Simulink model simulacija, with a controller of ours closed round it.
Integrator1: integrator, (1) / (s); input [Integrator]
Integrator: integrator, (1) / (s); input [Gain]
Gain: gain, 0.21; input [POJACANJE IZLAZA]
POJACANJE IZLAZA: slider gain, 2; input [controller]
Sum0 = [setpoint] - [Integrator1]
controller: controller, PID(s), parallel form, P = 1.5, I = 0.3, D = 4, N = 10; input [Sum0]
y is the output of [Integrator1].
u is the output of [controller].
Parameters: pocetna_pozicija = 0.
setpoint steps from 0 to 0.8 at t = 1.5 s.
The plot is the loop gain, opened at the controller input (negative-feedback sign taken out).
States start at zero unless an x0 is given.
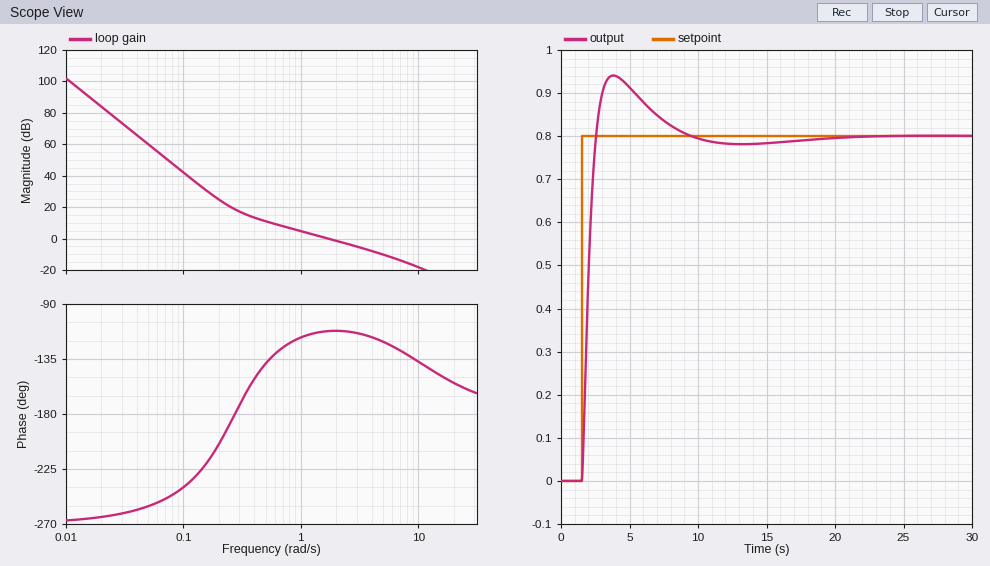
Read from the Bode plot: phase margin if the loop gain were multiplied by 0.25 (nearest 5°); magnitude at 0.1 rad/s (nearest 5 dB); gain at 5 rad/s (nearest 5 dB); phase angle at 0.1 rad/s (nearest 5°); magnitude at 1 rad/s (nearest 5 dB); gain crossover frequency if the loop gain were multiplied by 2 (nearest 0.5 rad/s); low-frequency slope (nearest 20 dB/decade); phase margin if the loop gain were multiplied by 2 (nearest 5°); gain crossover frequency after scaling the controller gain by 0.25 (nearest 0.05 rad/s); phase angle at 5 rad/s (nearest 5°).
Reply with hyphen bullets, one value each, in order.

- 35°
- 40 dB
- -10 dB
- -240°
- 5 dB
- 3.5 rad/s
- -60 dB/decade
- 65°
- 0.45 rad/s
- -120°
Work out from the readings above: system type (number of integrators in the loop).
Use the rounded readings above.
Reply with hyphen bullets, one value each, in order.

- 3
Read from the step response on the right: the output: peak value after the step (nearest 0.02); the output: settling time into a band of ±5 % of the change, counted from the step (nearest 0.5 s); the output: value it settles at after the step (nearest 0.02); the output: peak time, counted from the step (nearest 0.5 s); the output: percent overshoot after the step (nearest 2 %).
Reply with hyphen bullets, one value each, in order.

- 0.94
- 6.0 s
- 0.80
- 2.5 s
- 18 %
